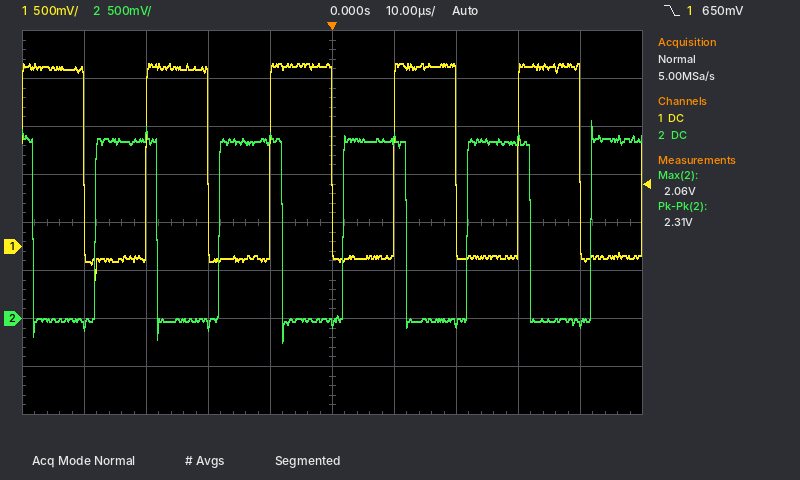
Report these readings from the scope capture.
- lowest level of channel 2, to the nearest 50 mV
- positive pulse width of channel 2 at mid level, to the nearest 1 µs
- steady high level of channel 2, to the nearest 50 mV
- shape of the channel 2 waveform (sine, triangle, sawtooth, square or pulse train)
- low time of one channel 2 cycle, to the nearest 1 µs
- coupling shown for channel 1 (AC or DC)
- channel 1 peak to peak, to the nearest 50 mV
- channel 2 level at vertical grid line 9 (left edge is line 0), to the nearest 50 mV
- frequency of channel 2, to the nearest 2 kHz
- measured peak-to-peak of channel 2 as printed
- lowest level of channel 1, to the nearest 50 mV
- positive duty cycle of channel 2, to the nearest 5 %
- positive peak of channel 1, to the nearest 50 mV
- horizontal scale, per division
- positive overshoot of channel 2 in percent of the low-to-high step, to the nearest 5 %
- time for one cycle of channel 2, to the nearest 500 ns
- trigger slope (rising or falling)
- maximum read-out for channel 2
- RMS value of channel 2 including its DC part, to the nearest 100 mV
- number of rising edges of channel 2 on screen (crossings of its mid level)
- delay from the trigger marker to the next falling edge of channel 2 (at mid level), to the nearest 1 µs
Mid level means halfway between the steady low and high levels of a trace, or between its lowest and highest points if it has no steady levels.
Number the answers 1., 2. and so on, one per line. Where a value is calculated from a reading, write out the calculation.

1. -250 mV
2. 10 µs
3. 1.85 V
4. square
5. 10 µs
6. DC
7. 1.90 V − (-350 mV) = 2.25 V
8. -50 mV
9. 1 / 20.0 µs ≈ 50 kHz
10. 2.31 V
11. -350 mV
12. 10 µs / 20.0 µs ≈ 50 %
13. 1.90 V
14. 10 µs
15. 10 %
16. 20.0 µs
17. falling
18. 2.06 V
19. √(0.5 × (1.85 V)² + 0.5 × (-250 mV)²) ≈ 1.3 V
20. 5
21. 12 µs
